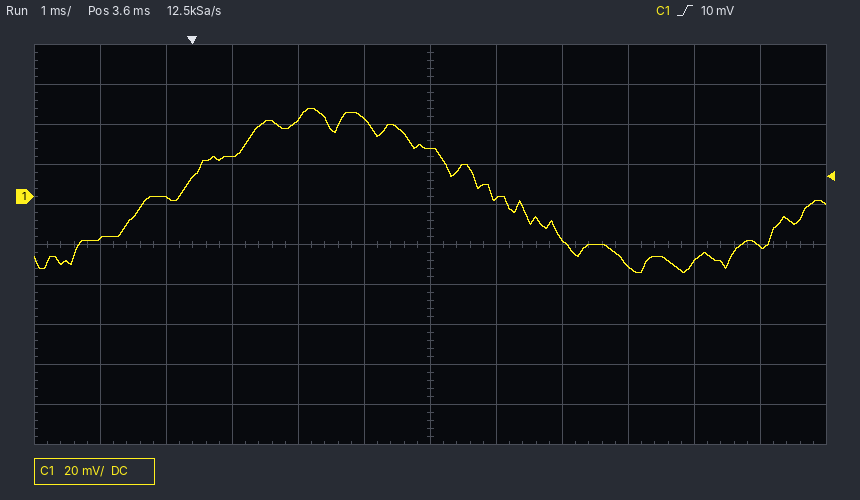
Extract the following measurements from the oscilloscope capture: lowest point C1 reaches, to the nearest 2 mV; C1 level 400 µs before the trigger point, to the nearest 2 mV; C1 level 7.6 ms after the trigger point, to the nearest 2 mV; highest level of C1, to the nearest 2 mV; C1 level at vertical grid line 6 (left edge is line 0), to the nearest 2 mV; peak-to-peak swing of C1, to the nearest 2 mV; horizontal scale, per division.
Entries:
-38 mV
0 mV
-32 mV
44 mV
24 mV
82 mV
1 ms
